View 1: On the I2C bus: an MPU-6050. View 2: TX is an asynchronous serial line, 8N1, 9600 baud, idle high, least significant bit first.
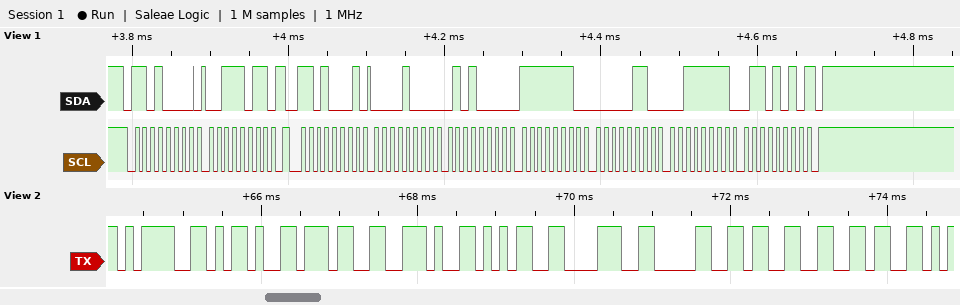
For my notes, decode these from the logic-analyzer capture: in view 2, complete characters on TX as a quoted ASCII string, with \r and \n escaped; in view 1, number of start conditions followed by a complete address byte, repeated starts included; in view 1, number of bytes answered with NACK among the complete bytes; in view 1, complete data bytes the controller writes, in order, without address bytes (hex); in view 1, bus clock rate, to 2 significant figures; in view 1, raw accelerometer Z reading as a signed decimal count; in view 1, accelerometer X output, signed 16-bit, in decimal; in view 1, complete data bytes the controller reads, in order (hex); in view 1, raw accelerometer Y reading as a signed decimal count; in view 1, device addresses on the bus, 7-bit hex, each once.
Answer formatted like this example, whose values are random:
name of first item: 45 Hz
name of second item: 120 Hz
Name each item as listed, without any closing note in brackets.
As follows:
in view 2, complete characters on TX as a quoted ASCII string, with \r and \n escaped: "=-7.58036"
in view 1, number of start conditions followed by a complete address byte, repeated starts included: 2
in view 1, number of bytes answered with NACK among the complete bytes: 1
in view 1, complete data bytes the controller writes, in order, without address bytes: 3B
in view 1, bus clock rate, to 2 significant figures: 100 kHz
in view 1, raw accelerometer Z reading as a signed decimal count: 16234
in view 1, accelerometer X output, signed 16-bit, in decimal: 2128
in view 1, complete data bytes the controller reads, in order: 08 50 FE 06 3F 6A
in view 1, raw accelerometer Y reading as a signed decimal count: -506
in view 1, device addresses on the bus, 7-bit hex, each once: 0x68
